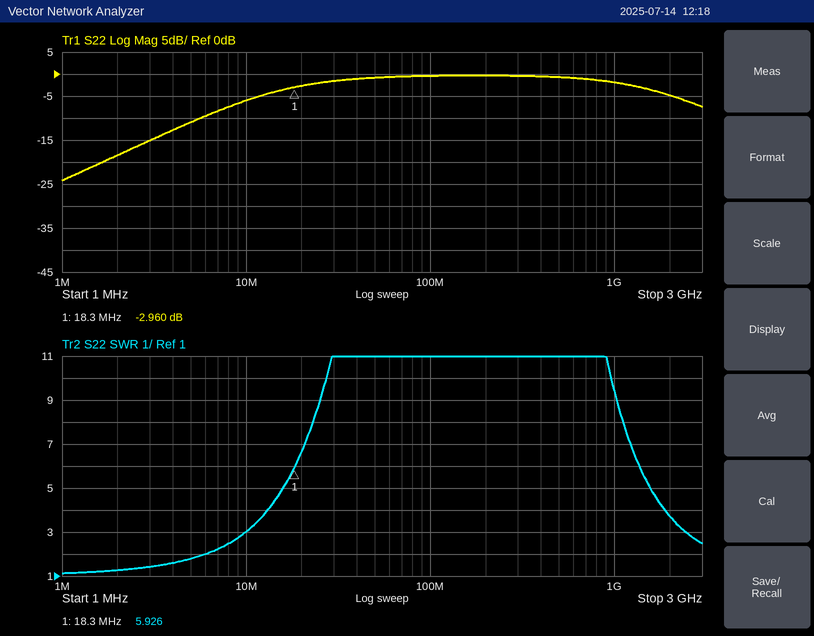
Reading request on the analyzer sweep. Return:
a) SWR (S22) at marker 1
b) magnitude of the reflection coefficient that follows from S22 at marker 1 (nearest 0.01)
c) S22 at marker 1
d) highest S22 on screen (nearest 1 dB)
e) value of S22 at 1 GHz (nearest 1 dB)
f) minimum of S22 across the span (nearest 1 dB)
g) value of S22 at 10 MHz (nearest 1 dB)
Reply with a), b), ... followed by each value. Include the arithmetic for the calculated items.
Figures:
a) 5.926
b) 10^(-2.96/20) ≈ 0.71
c) -2.960 dB
d) 0 dB
e) -2 dB
f) -24 dB
g) -6 dB
